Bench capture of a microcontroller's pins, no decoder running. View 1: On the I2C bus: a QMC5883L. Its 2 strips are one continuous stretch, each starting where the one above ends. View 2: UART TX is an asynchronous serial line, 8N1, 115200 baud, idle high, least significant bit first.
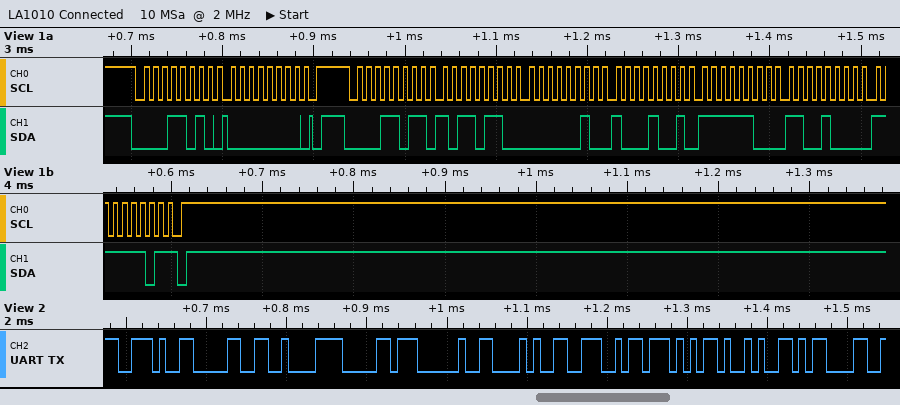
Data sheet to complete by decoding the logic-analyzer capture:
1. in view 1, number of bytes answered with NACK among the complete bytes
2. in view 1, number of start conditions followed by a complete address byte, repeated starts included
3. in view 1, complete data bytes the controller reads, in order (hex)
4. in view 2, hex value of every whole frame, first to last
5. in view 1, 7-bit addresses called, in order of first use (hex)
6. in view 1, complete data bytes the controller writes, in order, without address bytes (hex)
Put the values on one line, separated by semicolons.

1; 2; B6 02 89 FC C8 FD; 2E 30 C2 B0 20 28 4E 57 29 0D; 0x0D; 00
